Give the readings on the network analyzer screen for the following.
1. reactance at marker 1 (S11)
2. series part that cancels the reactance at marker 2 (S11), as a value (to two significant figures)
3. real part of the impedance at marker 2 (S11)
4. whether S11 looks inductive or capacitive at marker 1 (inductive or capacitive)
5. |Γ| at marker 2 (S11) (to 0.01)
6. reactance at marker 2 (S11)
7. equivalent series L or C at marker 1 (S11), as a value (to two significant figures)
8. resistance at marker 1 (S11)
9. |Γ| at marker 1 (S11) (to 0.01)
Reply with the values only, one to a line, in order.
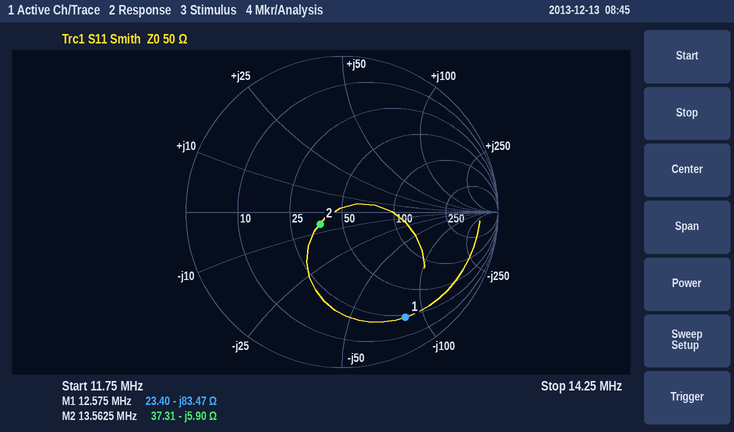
-83.47 Ω
69 nH
37.31 Ω
capacitive
0.16
-5.90 Ω
150 pF
23.40 Ω
0.79
